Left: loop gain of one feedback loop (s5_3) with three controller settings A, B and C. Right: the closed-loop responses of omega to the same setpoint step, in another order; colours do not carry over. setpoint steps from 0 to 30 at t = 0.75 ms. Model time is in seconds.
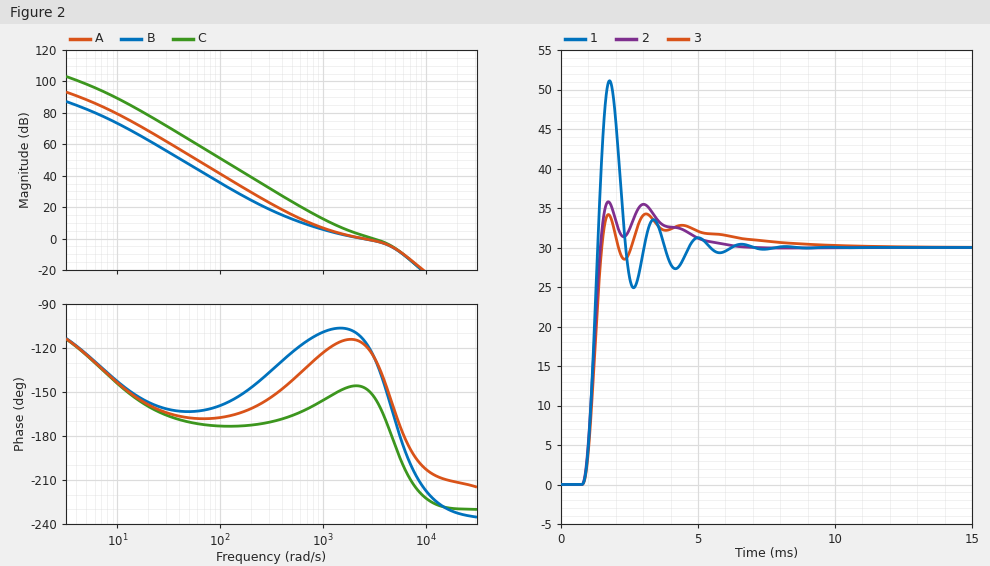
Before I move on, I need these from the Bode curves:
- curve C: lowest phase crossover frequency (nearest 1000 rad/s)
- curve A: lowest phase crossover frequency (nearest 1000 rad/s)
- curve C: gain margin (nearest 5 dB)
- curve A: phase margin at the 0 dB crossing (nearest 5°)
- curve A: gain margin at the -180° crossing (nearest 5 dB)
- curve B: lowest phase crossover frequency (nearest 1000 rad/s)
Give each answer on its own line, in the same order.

5000 rad/s
6000 rad/s
5 dB
65°
10 dB
6000 rad/s
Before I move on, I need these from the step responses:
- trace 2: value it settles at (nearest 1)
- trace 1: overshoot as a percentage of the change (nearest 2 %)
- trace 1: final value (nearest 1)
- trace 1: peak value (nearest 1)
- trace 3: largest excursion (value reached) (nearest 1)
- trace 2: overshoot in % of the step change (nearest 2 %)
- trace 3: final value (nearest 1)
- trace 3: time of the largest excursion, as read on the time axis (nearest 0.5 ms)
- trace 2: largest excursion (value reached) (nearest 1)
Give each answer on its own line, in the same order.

30
70 %
30
51
34
20 %
30
3.0 ms
36
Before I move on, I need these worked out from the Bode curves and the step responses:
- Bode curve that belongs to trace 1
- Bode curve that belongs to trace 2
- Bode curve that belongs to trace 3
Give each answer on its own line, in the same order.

C
A
B
